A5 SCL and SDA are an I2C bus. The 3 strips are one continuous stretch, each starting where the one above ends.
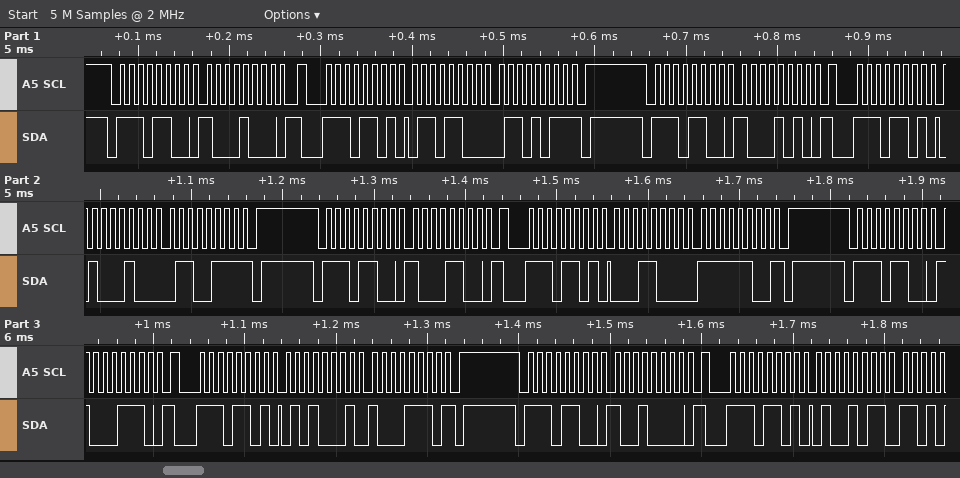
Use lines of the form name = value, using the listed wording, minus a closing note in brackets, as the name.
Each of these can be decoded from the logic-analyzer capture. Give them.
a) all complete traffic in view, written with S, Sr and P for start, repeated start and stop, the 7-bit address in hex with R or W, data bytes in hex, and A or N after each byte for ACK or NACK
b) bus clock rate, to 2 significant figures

all complete traffic in view, written with S, Sr and P for start, repeated start and stop, the 7-bit address in hex with R or W, data bytes in hex, and A or N after each byte for ACK or NACK = S 76W A 88 A Sr 76R A 6C A 6B N P S 76W A 8A A Sr 76R A 44 A 67 N P S 76W A 8C A Sr 76R A 18 A FC N P S 76W A 8E A Sr 76R A 51 A 8E N P S 76W A 90 A Sr 76R A 4B A
bus clock rate, to 2 significant figures = 100 kHz
